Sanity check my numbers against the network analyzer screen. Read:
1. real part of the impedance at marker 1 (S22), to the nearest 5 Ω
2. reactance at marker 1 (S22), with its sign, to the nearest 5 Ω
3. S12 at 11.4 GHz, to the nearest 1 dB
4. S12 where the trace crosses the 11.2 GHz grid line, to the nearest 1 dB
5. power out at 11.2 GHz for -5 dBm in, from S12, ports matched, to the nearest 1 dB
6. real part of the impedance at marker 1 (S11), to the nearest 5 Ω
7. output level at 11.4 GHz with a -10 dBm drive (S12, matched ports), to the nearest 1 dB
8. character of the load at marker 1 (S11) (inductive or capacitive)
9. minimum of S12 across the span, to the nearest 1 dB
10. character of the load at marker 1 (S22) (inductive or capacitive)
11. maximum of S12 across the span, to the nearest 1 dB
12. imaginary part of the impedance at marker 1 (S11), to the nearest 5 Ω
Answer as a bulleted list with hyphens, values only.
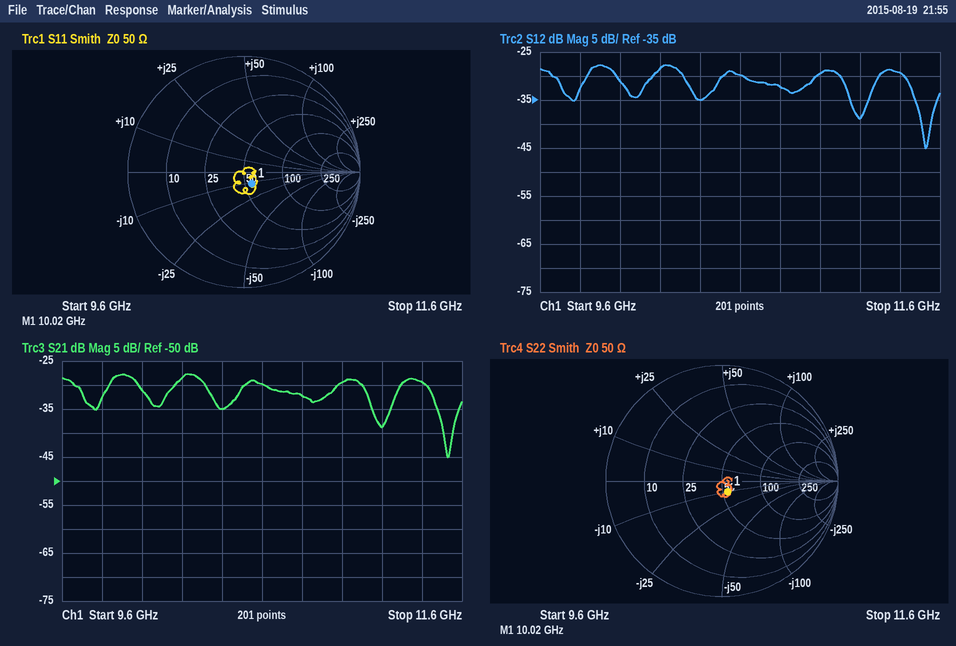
- 55 Ω
- -10 Ω
- -29 dB
- -39 dB
- -44 dBm
- 55 Ω
- -39 dBm
- capacitive
- -45 dB
- capacitive
- -28 dB
- -10 Ω
